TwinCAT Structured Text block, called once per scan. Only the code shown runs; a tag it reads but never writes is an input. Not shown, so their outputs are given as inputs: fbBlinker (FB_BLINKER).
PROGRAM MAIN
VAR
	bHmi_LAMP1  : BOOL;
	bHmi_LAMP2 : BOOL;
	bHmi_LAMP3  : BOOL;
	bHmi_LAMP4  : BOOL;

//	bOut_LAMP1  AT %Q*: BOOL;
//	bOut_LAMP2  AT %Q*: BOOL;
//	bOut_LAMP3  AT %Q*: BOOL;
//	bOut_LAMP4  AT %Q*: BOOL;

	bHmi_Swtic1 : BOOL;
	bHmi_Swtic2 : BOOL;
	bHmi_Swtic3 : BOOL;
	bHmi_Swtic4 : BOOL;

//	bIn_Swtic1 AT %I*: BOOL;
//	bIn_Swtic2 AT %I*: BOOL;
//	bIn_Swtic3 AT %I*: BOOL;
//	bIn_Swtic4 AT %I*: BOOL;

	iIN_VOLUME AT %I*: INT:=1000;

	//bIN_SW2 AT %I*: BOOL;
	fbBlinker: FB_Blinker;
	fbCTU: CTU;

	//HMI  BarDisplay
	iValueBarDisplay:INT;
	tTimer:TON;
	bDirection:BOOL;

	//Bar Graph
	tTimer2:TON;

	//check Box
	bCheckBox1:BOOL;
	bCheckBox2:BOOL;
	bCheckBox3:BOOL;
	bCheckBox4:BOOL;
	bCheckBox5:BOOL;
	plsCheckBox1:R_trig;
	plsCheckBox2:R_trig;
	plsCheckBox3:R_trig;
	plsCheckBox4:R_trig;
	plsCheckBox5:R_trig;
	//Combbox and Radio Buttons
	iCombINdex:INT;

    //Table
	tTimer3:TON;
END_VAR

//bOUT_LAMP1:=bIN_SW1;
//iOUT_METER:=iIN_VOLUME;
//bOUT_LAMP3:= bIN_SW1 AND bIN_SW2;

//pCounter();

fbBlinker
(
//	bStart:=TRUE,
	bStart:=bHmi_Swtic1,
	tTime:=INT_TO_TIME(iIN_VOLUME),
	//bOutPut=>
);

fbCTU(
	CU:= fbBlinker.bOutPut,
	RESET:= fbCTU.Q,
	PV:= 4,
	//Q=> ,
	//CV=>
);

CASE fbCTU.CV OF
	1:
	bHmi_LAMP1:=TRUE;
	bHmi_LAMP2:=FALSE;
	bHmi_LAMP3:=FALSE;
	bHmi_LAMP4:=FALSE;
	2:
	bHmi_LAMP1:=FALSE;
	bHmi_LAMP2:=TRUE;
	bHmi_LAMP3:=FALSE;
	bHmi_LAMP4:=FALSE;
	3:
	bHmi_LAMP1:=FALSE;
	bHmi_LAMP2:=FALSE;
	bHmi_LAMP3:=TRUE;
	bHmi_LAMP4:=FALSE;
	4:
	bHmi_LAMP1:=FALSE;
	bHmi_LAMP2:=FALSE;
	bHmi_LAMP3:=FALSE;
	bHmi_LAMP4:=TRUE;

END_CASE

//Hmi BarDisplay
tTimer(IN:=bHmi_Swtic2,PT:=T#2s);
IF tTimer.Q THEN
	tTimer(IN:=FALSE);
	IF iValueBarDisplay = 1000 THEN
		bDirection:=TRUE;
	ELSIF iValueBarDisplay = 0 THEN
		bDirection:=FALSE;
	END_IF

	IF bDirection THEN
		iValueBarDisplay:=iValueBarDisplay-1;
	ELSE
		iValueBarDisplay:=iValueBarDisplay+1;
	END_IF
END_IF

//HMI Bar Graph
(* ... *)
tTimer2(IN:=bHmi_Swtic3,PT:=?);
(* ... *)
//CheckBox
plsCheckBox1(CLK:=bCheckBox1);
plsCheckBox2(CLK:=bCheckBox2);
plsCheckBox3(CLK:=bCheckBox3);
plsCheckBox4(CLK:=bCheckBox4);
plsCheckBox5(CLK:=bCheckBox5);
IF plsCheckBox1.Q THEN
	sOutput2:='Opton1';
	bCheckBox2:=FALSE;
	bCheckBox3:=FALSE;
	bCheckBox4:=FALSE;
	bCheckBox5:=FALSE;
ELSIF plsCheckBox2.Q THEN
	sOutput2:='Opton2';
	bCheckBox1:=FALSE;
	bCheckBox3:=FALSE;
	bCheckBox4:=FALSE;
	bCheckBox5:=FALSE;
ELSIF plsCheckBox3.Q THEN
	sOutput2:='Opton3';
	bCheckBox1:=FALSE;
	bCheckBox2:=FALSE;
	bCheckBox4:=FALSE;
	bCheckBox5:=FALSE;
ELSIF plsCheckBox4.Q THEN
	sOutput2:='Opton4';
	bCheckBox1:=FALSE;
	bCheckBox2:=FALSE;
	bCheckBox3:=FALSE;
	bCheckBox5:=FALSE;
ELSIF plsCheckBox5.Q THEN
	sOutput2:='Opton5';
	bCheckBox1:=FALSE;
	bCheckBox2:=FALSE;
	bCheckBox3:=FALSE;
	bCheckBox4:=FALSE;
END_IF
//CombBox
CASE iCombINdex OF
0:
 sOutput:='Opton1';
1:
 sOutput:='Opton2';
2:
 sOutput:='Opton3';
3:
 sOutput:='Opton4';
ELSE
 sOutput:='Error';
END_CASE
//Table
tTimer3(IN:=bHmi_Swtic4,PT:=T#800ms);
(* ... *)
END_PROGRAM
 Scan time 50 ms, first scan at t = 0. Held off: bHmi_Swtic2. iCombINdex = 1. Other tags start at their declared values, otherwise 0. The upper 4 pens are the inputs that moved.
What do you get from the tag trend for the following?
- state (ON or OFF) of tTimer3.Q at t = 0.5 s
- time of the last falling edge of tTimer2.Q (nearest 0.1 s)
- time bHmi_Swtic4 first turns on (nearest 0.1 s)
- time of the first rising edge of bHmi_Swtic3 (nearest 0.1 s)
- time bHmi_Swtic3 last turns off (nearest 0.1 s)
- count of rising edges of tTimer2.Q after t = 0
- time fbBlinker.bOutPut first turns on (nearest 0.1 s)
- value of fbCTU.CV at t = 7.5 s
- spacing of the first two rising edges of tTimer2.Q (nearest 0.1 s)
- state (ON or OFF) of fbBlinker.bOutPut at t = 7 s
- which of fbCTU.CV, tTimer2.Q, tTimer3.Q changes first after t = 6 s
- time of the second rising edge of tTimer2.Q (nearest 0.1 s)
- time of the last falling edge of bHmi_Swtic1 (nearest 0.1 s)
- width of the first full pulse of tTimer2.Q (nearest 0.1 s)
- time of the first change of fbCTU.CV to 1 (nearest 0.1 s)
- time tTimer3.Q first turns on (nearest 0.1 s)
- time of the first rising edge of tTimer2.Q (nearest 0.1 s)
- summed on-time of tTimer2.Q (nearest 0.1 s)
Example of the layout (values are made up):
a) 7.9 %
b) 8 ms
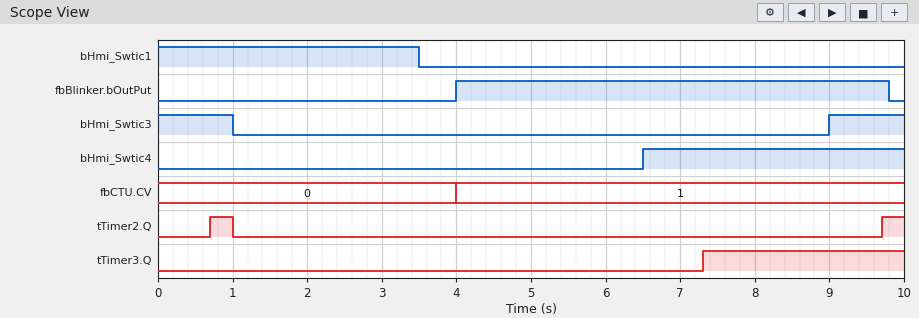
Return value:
a) OFF
b) 1.0 s
c) 6.5 s
d) 9.0 s
e) 1.0 s
f) 2
g) 4.0 s
h) 1
i) 9.0 s
j) ON
k) tTimer3.Q
l) 9.7 s
m) 3.5 s
n) 0.3 s
o) 4.0 s
p) 7.3 s
q) 0.7 s
r) 0.6 s
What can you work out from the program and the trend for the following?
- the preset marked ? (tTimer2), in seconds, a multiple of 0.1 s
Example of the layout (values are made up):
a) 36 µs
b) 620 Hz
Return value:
a) 0.7 s
